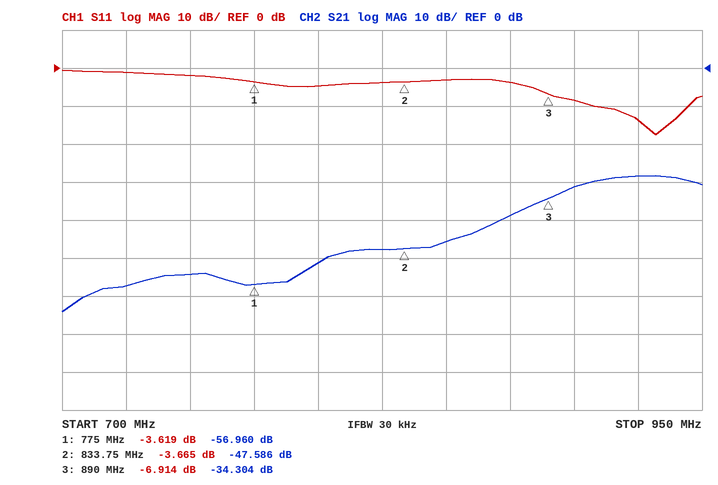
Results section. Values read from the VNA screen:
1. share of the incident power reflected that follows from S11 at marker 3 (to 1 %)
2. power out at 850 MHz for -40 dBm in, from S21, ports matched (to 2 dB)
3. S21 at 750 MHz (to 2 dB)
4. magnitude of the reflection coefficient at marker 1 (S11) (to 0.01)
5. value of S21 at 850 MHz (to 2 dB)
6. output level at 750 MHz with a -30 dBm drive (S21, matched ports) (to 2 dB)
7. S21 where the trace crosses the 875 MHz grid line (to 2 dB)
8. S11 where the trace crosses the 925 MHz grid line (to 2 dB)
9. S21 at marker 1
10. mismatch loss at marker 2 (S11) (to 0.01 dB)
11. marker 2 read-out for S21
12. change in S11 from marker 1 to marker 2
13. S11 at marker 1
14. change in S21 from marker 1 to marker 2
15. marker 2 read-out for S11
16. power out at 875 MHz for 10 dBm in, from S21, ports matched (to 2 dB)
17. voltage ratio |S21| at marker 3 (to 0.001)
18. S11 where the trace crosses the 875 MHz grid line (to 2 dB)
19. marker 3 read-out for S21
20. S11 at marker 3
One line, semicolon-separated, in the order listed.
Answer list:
20 %; -86 dBm; -54 dB; 0.66; -46 dB; -84 dBm; -38 dB; -14 dB; -56.960 dB; 2.44 dB; -47.586 dB; -0.046 dB; -3.619 dB; 9.374 dB; -3.665 dB; -28 dBm; 0.019; -4 dB; -34.304 dB; -6.914 dB
